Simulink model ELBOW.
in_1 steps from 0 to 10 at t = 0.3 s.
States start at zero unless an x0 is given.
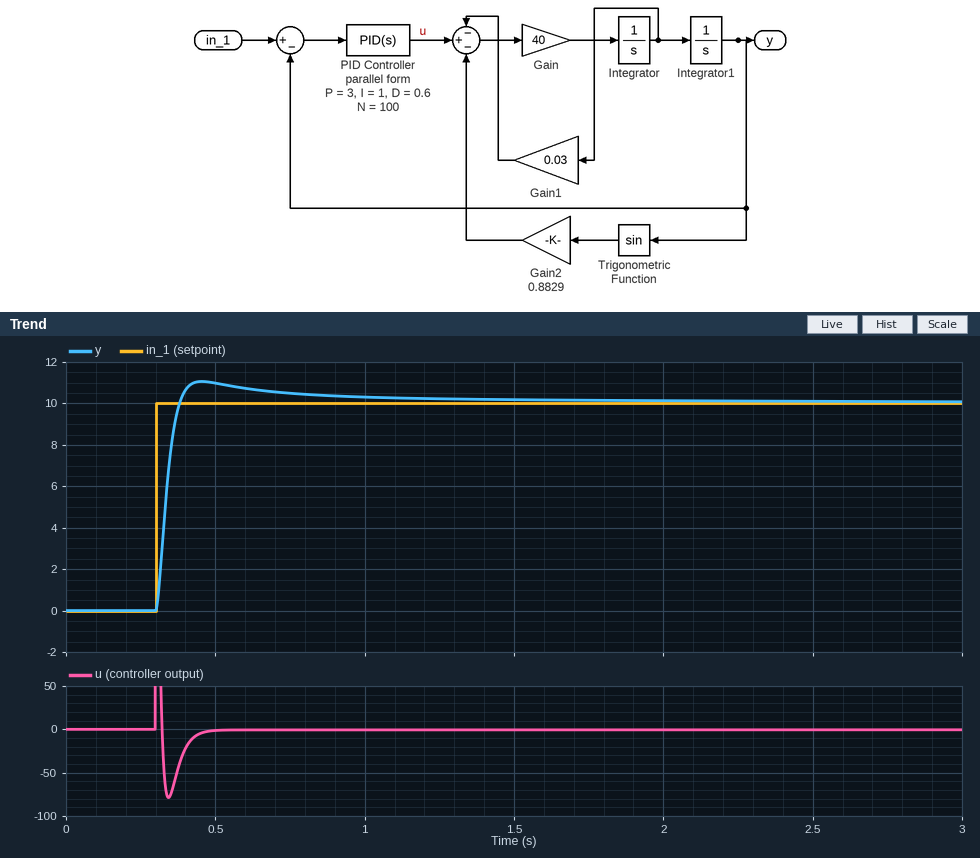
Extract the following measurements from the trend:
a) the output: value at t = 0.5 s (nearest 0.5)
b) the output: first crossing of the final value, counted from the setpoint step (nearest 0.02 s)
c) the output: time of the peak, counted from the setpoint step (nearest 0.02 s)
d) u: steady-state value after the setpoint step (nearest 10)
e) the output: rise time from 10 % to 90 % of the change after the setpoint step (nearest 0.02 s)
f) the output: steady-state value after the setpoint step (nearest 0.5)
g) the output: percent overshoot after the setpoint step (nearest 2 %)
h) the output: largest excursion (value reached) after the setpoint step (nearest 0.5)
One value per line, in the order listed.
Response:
11.0
0.08 s
0.16 s
0
0.06 s
10.0
10 %
11.0
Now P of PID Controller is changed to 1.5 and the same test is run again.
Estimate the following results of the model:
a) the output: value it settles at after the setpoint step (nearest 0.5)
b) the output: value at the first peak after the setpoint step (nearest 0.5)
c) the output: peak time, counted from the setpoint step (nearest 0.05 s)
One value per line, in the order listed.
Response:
10.0
10.5
0.60 s
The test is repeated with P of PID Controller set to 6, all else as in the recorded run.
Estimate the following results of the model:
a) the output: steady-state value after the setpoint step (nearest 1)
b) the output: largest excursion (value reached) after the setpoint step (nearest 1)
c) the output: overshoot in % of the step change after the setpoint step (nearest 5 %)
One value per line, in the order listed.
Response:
10
12
20 %
